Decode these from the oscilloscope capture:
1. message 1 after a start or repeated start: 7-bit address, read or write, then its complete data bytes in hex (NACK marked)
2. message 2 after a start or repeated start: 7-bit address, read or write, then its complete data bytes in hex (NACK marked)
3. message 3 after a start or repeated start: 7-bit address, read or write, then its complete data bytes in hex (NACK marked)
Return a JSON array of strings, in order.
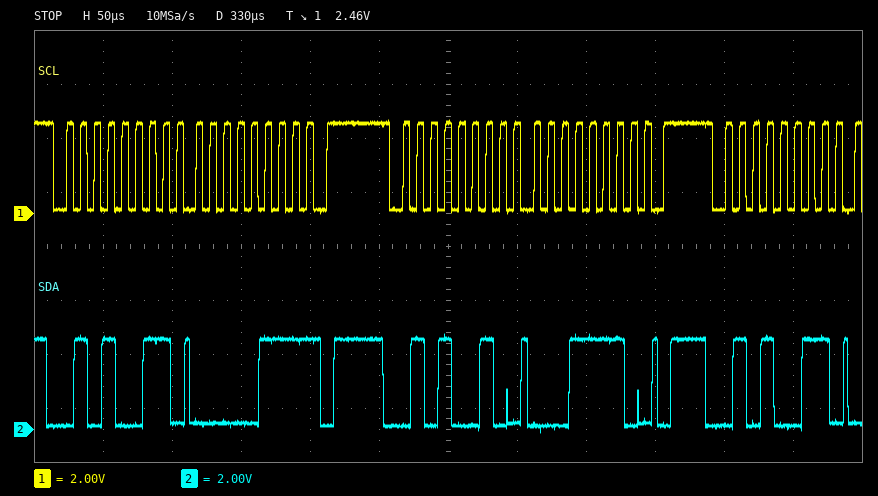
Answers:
["0x29 read: 07 NACK", "0x29 write: 1E", "0x29 read"]
